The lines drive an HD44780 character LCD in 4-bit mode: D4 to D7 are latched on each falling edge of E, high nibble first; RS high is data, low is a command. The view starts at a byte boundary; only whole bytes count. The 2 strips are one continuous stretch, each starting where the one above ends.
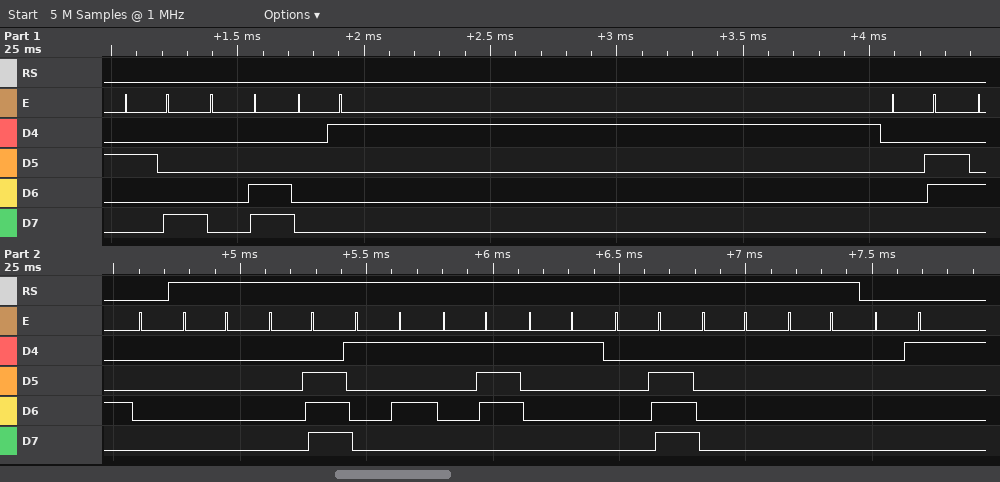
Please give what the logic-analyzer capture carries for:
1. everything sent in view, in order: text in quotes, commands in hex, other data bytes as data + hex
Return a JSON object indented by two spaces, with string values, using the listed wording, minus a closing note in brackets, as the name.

{
  "everything sent in view, in order: text in quotes, commands in hex, other data bytes as data + hex": "0x28 0x0C 0x01 0x06 0x40 data 00 0E 15 17 11 0E 00 00 0x01"
}
